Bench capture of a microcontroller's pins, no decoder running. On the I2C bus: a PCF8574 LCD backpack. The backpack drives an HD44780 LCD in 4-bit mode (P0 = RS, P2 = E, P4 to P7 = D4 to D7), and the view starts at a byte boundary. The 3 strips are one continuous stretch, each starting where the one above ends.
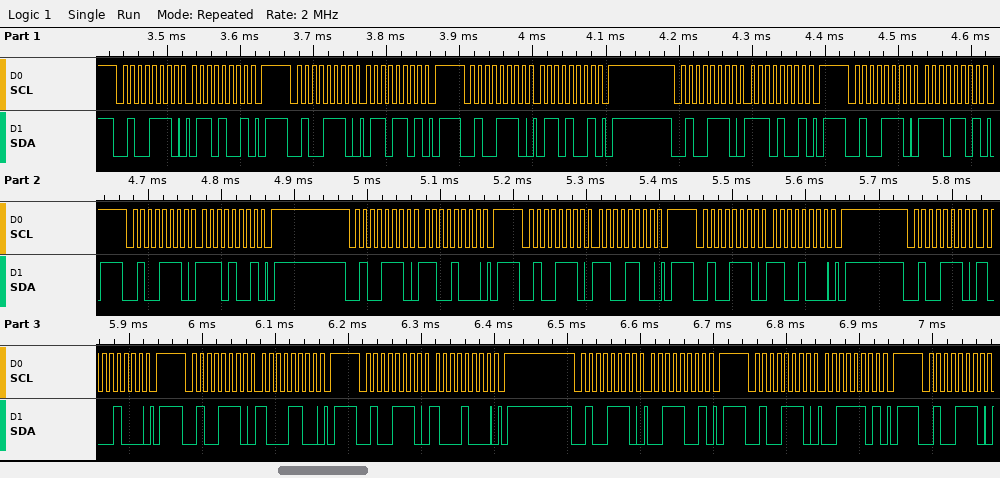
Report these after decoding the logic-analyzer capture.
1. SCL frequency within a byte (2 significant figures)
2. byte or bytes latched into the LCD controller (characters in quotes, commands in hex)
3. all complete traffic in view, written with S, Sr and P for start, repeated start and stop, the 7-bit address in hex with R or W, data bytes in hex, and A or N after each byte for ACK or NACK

100 kHz
'n' 0xC8
S 27W A 69 A P S 27W A 6D A P S 27W A 69 A P S 27W A E9 A P S 27W A ED A P S 27W A E9 A P S 27W A C8 A P S 27W A CC A P S 27W A C8 A P S 27W A 88 A P S 27W A 8C A P S 27W A 88 A P S 27W A 39 A P S 27W A 3D A P S 27W A
